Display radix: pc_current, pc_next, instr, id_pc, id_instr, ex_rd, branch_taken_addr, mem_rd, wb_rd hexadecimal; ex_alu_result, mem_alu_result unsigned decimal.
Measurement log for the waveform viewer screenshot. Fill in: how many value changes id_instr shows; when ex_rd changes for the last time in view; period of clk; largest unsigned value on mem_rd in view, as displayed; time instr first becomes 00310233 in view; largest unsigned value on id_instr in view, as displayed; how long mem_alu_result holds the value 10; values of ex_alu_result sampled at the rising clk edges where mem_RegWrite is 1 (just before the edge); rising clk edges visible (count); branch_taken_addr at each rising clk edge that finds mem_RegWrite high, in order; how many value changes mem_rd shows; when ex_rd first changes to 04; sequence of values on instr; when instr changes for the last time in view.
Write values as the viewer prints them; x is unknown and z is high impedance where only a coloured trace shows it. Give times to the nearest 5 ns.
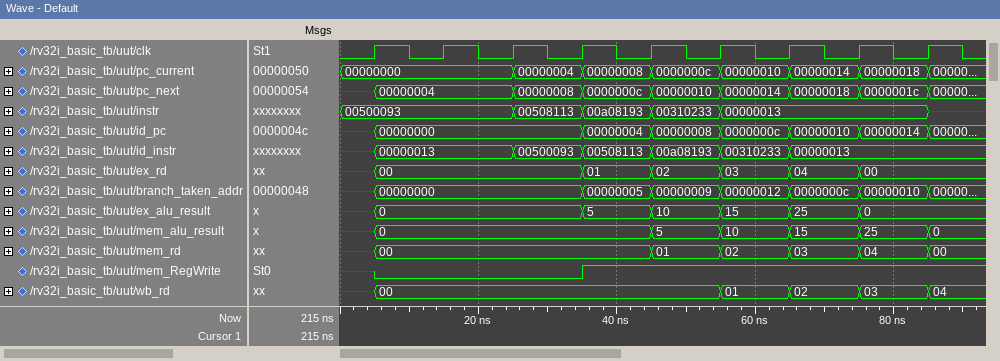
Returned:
6
75 ns
10 ns
04
45 ns
00a08193
10 ns
5, 10, 15, 25, 0
9
00000005, 00000009, 00000012, 0000000c, 00000010
6
65 ns
00500093, 00508113, 00a08193, 00310233, 00000013, x
85 ns
